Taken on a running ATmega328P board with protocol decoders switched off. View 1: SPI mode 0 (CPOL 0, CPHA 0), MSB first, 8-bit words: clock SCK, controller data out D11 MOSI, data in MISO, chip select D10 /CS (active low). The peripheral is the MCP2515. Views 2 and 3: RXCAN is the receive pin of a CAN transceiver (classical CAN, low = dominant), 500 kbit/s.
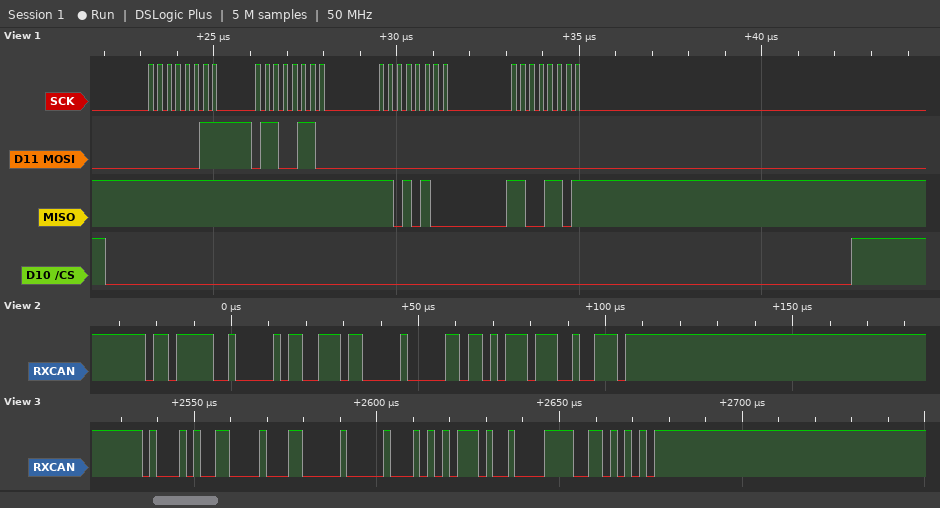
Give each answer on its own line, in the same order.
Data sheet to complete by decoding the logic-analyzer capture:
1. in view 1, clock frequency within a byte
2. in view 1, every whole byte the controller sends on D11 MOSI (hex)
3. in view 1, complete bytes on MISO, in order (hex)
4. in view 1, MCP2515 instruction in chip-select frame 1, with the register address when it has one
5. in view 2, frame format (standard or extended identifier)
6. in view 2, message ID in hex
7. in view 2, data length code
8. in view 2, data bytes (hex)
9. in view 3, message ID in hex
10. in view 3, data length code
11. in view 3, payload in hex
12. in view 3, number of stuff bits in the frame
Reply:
4 MHz
03 66 00 00
FF FF D4 CD
READ 0x66
standard
0x6FA
3
3B 00 2D
0x453
4
60 00 AB A4
2
